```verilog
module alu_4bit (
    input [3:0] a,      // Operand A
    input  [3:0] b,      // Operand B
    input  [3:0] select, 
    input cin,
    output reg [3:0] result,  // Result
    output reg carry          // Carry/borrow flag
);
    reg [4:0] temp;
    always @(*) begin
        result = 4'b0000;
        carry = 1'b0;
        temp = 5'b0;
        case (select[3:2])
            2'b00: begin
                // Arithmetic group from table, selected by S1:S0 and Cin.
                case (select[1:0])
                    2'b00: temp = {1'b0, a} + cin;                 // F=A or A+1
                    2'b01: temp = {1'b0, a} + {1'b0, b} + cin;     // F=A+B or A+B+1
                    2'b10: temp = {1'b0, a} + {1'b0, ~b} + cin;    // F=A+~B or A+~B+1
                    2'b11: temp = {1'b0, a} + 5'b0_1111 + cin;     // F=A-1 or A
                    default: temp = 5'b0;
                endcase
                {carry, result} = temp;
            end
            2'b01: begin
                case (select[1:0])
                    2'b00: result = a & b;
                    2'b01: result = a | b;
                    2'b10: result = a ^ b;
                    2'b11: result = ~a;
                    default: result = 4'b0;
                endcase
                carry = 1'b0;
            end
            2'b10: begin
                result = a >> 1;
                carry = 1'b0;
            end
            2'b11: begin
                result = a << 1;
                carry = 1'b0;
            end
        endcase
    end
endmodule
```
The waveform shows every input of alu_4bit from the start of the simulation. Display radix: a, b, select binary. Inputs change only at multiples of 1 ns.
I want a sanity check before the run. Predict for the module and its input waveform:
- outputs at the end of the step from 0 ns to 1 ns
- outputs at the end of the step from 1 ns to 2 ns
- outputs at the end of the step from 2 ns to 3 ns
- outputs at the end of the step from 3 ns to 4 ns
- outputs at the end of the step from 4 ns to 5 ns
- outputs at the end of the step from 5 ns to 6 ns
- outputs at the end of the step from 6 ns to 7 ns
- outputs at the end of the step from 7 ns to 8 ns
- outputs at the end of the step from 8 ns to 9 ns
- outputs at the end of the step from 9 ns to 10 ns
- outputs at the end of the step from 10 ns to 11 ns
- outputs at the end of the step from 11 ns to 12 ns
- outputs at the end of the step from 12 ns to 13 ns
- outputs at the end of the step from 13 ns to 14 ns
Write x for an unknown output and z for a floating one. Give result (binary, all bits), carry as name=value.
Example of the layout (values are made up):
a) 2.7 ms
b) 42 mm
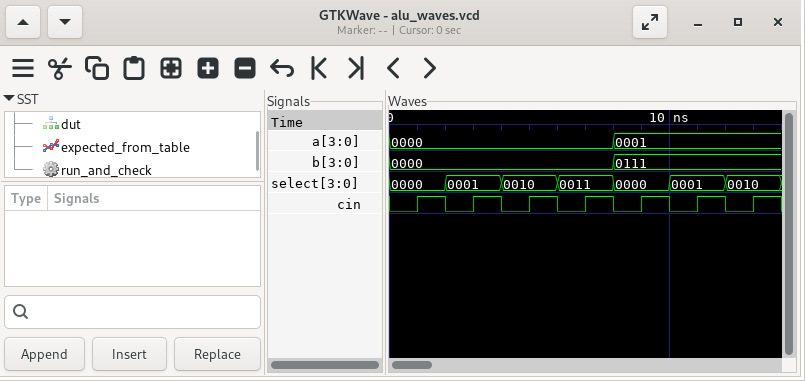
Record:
a) result=0000, carry=0
b) result=0001, carry=0
c) result=0000, carry=0
d) result=0001, carry=0
e) result=1111, carry=0
f) result=0000, carry=1
g) result=1111, carry=0
h) result=0000, carry=1
i) result=0001, carry=0
j) result=0010, carry=0
k) result=1000, carry=0
l) result=1001, carry=0
m) result=1001, carry=0
n) result=1010, carry=0
